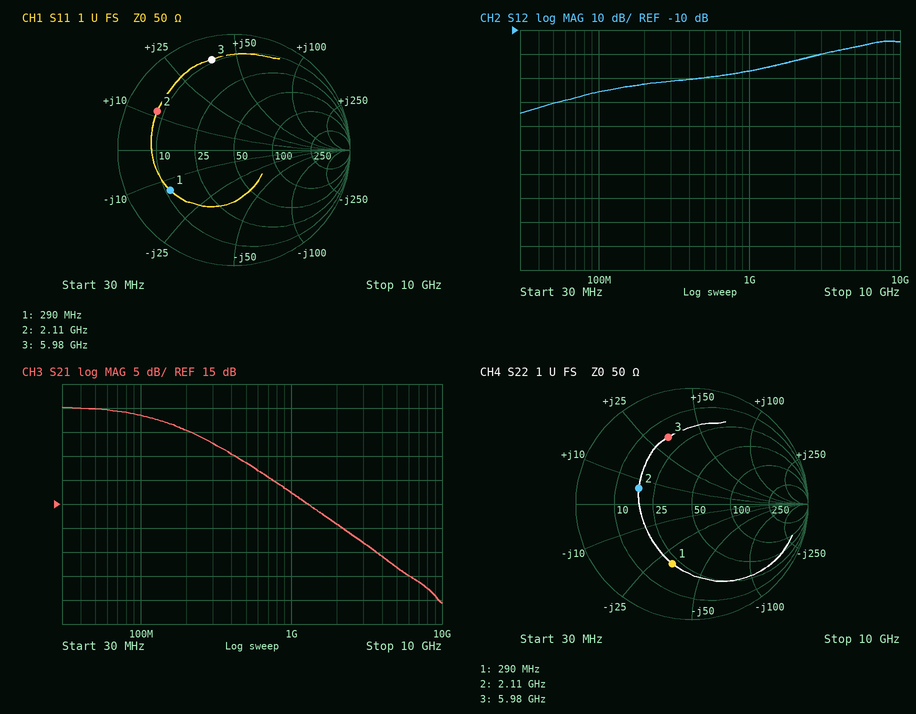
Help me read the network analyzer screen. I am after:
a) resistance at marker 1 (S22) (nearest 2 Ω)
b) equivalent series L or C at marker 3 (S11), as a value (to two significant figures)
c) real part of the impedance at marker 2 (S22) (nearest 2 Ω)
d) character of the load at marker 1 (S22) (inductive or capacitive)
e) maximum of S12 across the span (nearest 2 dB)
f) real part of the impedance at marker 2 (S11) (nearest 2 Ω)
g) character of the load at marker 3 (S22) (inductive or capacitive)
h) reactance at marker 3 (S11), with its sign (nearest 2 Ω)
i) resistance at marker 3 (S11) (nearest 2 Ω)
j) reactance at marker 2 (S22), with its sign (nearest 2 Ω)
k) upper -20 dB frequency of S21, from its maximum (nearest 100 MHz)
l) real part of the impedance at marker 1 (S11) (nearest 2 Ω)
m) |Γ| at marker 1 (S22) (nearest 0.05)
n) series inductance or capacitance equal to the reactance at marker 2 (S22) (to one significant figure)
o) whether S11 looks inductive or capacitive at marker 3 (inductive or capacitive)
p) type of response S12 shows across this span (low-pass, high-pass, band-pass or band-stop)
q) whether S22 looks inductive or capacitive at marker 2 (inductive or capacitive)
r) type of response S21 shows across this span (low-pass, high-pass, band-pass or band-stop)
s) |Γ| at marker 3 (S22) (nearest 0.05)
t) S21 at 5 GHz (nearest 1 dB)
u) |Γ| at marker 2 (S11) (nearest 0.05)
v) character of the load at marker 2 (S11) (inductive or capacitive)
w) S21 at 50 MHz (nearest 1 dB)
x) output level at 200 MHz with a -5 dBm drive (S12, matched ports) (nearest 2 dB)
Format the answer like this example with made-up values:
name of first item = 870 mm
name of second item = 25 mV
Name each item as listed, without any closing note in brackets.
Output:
resistance at marker 1 (S22) = 22 Ω
equivalent series L or C at marker 3 (S11), as a value = 1.0 nH
real part of the impedance at marker 2 (S22) = 18 Ω
character of the load at marker 1 (S22) = capacitive
maximum of S12 across the span = -14 dB
real part of the impedance at marker 2 (S11) = 8 Ω
character of the load at marker 3 (S22) = inductive
reactance at marker 3 (S11), with its sign = +38 Ω
resistance at marker 3 (S11) = 8 Ω
reactance at marker 2 (S22), with its sign = +6 Ω
upper -20 dB frequency of S21, from its maximum = 1.3 GHz
real part of the impedance at marker 1 (S11) = 12 Ω
|Γ| at marker 1 (S22) = 0.55
series inductance or capacitance equal to the reactance at marker 2 (S22) = 500 pH
whether S11 looks inductive or capacitive at marker 3 = inductive
type of response S12 shows across this span = high-pass
whether S22 looks inductive or capacitive at marker 2 = inductive
type of response S21 shows across this span = low-pass
|Γ| at marker 3 (S22) = 0.60
S21 at 5 GHz = 2 dB
|Γ| at marker 2 (S11) = 0.75
character of the load at marker 2 (S11) = inductive
S21 at 50 MHz = 35 dB
output level at 200 MHz with a -5 dBm drive (S12, matched ports) = -38 dBm
